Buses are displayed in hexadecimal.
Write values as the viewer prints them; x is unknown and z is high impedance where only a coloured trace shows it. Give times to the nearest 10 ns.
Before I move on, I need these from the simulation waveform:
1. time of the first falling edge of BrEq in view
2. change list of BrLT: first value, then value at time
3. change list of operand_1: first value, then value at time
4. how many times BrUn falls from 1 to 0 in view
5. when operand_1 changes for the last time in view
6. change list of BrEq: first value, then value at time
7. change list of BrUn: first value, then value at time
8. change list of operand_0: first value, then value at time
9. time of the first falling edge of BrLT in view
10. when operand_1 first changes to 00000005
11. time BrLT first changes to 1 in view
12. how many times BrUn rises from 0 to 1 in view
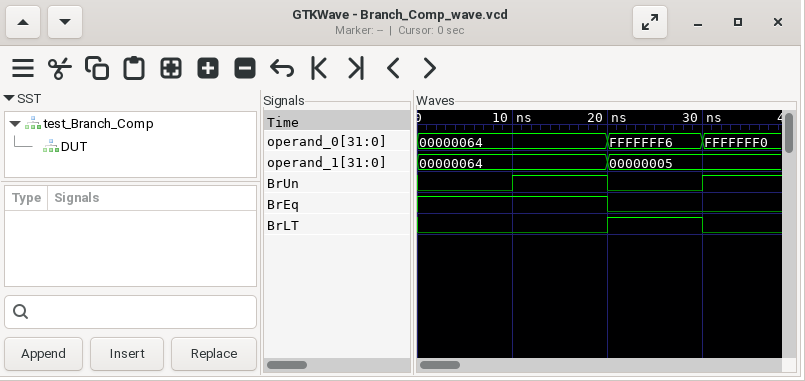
20 ns
0, 1 at 20 ns, 0 at 30 ns
00000064, 00000005 at 20 ns
1
20 ns
1, 0 at 20 ns
0, 1 at 10 ns, 0 at 20 ns, 1 at 30 ns
00000064, FFFFFFF6 at 20 ns, FFFFFFF0 at 30 ns
30 ns
20 ns
20 ns
2
